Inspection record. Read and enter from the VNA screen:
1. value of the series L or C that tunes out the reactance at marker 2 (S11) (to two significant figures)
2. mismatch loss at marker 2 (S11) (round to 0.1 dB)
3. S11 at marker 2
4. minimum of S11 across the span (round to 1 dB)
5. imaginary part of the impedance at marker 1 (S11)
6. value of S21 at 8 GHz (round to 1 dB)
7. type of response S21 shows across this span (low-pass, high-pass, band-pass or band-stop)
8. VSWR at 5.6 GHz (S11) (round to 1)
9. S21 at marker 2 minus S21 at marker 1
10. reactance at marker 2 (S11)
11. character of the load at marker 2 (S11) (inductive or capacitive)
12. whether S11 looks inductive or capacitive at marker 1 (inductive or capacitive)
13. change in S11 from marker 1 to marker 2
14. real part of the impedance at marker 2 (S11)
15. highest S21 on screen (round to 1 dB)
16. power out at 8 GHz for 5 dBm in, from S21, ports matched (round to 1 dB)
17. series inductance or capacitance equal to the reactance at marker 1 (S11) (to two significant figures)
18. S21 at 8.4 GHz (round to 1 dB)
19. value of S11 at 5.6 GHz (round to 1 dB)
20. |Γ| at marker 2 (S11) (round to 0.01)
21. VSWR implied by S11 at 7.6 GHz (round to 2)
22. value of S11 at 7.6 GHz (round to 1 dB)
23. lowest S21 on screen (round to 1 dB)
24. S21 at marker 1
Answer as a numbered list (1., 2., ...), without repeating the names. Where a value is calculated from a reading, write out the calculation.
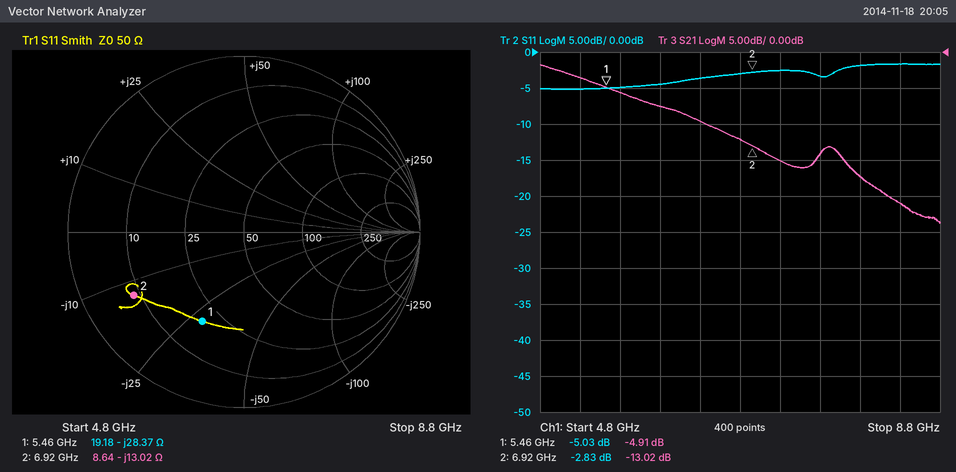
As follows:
1. L = 13.02 Ω/(2π × 6.92 GHz) ≈ 299 pH, so 300 pH to two significant figures
2. −10 log10(1 − 10^(-2.83/10)) ≈ 3.2 dB
3. -2.83 dB
4. -5 dB
5. -28.37 Ω
6. -17 dB
7. low-pass
8. |Γ| = 10^(-5/20) = 0.5623; VSWR = (1 + 0.5623)/(1 − 0.5623) ≈ 4
9. -13.02 − (-4.91) = -8.11 dB
10. -13.02 Ω
11. capacitive
12. capacitive
13. -2.83 − (-5.03) = 2.20 dB
14. 8.64 Ω
15. -2 dB
16. 5 dBm + (-17 dB) = -12 dBm
17. C = 1/(2π × 5.46 GHz × 28.37 Ω) ≈ 1.0 pF
18. -21 dB
19. -5 dB
20. 0.72
21. |Γ| = 10^(-3/20) = 0.7079; VSWR = (1 + 0.7079)/(1 − 0.7079) ≈ 6
22. -3 dB
23. -24 dB
24. -4.91 dB
